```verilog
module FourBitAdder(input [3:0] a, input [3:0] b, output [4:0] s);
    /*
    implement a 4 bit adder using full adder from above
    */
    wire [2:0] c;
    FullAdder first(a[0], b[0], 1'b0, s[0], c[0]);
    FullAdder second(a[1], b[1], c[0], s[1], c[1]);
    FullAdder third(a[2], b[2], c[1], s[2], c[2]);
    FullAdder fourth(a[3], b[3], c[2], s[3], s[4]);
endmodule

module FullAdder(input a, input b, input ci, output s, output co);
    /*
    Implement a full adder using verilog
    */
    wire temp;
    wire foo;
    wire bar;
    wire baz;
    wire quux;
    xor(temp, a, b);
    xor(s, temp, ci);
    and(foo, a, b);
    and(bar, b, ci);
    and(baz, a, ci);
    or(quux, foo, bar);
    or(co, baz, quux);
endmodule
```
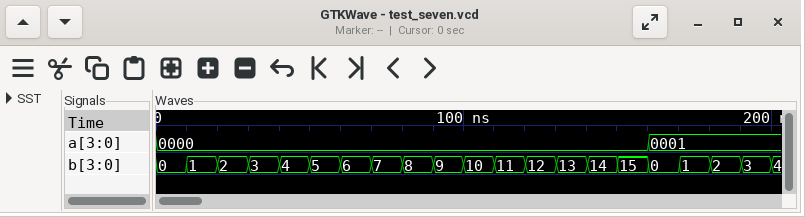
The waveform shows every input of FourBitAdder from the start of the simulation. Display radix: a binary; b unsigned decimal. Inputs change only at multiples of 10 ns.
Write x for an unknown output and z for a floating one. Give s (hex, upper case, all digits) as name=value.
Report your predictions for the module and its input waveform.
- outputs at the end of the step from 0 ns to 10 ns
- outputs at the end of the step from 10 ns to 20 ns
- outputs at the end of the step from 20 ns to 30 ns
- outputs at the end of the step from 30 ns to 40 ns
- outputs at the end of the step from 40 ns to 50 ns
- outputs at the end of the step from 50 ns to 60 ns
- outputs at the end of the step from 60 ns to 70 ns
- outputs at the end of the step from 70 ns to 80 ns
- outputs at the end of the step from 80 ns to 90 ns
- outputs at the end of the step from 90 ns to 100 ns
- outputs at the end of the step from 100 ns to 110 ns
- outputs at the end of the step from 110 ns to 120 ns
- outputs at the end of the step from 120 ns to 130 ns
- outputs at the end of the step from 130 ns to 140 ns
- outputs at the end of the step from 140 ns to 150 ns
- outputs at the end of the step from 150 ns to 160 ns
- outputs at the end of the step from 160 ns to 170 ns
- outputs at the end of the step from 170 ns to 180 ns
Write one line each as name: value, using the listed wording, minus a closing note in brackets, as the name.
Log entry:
outputs at the end of the step from 0 ns to 10 ns: s=00
outputs at the end of the step from 10 ns to 20 ns: s=01
outputs at the end of the step from 20 ns to 30 ns: s=02
outputs at the end of the step from 30 ns to 40 ns: s=03
outputs at the end of the step from 40 ns to 50 ns: s=04
outputs at the end of the step from 50 ns to 60 ns: s=05
outputs at the end of the step from 60 ns to 70 ns: s=06
outputs at the end of the step from 70 ns to 80 ns: s=07
outputs at the end of the step from 80 ns to 90 ns: s=08
outputs at the end of the step from 90 ns to 100 ns: s=09
outputs at the end of the step from 100 ns to 110 ns: s=0A
outputs at the end of the step from 110 ns to 120 ns: s=0B
outputs at the end of the step from 120 ns to 130 ns: s=0C
outputs at the end of the step from 130 ns to 140 ns: s=0D
outputs at the end of the step from 140 ns to 150 ns: s=0E
outputs at the end of the step from 150 ns to 160 ns: s=0F
outputs at the end of the step from 160 ns to 170 ns: s=01
outputs at the end of the step from 170 ns to 180 ns: s=02
